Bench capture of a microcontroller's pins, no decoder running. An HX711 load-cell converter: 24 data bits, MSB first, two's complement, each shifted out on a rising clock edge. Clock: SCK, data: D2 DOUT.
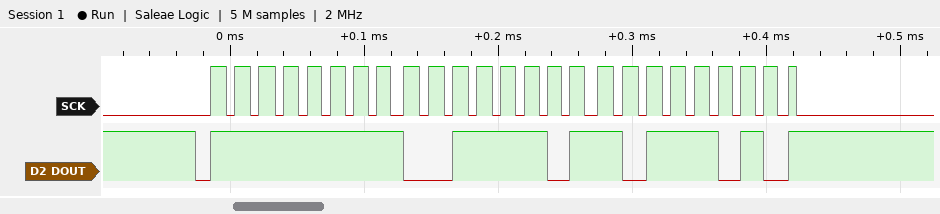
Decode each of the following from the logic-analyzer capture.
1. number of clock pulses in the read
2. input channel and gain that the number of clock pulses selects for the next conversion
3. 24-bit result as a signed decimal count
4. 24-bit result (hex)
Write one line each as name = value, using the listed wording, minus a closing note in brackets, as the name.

number of clock pulses in the read = 25
input channel and gain that the number of clock pulses selects for the next conversion = channel A, gain 128
24-bit result as a signed decimal count = -49734
24-bit result = 0xFF3DBA
